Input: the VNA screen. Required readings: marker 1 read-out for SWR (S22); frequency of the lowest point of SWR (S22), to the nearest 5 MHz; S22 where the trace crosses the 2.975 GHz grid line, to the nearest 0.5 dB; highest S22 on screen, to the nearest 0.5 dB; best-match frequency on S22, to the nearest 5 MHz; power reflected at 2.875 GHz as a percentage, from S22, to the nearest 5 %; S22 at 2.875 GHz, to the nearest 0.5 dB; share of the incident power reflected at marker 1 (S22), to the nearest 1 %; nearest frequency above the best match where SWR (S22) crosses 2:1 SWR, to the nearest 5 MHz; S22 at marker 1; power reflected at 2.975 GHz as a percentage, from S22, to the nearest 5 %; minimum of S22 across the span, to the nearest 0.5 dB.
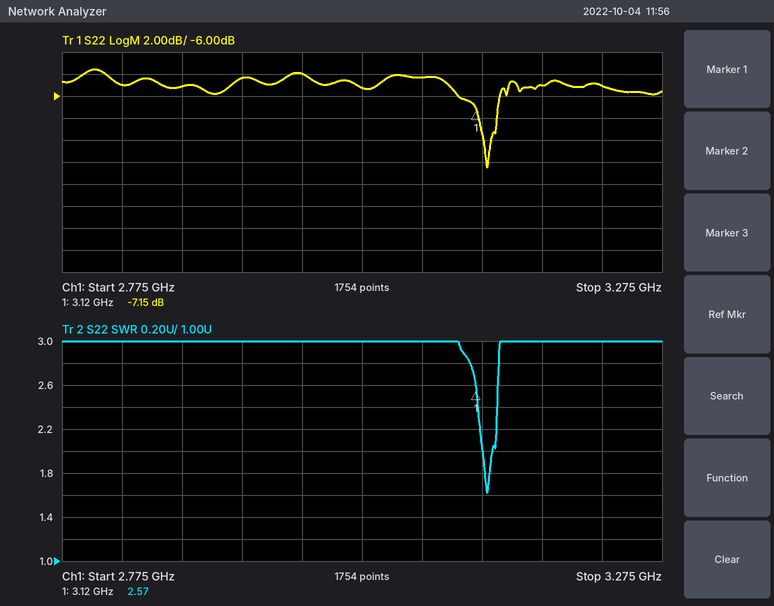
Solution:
2.57
3.130 GHz
-4.0 dB
-3.5 dB
3.130 GHz
30 %
-5.0 dB
19 %
3.135 GHz
-7.15 dB
40 %
-12.5 dB
